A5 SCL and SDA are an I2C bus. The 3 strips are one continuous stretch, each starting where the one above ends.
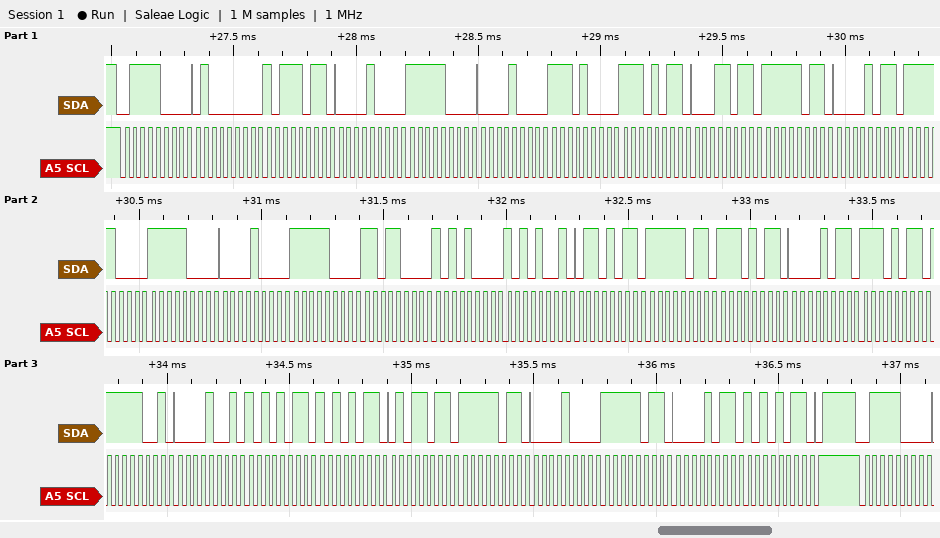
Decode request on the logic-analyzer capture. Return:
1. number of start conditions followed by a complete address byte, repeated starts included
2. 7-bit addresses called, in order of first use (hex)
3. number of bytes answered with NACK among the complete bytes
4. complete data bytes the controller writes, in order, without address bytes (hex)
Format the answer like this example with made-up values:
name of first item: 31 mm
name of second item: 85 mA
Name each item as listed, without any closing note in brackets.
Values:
number of start conditions followed by a complete address byte, repeated starts included: 2
7-bit addresses called, in order of first use: 0x3C
number of bytes answered with NACK among the complete bytes: 0
complete data bytes the controller writes, in order, without address bytes: 40 BB 08 F8 08 E8 EB 1B FB 0B F8 F8 08 F8 D8 A8 A9 6B FB EB 0B EB F9 09 AB AB 5B FB 08 FB 0B AB
